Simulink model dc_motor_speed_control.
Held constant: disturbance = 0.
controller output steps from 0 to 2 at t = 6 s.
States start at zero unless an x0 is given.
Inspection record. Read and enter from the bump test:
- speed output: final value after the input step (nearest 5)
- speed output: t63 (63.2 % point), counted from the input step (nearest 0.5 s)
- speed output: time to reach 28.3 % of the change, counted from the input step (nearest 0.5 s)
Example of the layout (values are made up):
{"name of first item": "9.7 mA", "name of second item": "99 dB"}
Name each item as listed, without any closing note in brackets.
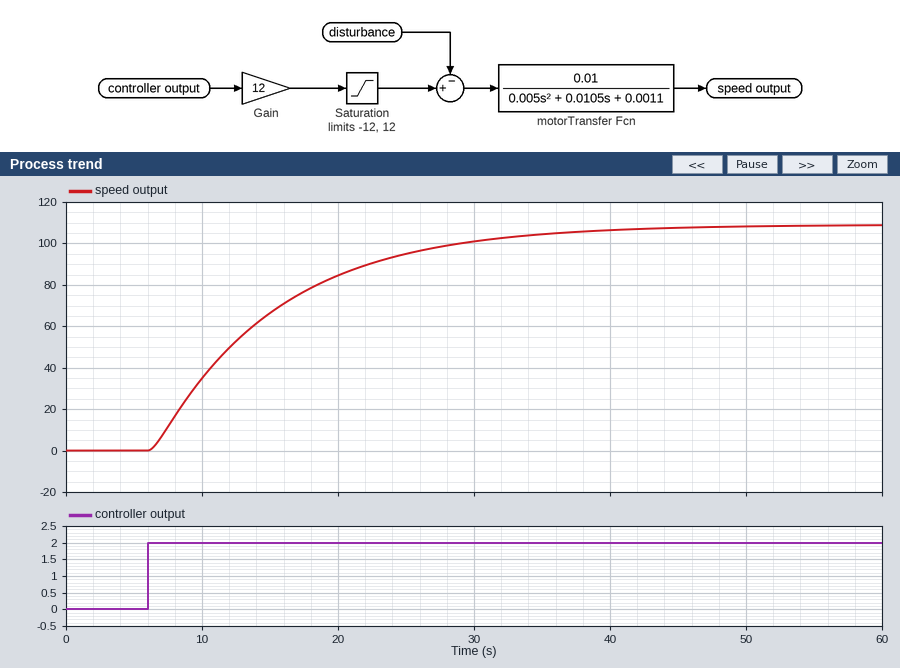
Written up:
{"speed output: final value after the input step": "110", "speed output: t63 (63.2 % point), counted from the input step": "9.5 s", "speed output: time to reach 28.3 % of the change, counted from the input step": "3.5 s"}
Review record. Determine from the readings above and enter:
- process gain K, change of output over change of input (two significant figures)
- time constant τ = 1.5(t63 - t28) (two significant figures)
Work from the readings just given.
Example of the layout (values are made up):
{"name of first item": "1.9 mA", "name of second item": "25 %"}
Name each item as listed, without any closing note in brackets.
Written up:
{"process gain K, change of output over change of input": "55", "time constant τ = 1.5(t63 - t28)": "9.0 s"}
